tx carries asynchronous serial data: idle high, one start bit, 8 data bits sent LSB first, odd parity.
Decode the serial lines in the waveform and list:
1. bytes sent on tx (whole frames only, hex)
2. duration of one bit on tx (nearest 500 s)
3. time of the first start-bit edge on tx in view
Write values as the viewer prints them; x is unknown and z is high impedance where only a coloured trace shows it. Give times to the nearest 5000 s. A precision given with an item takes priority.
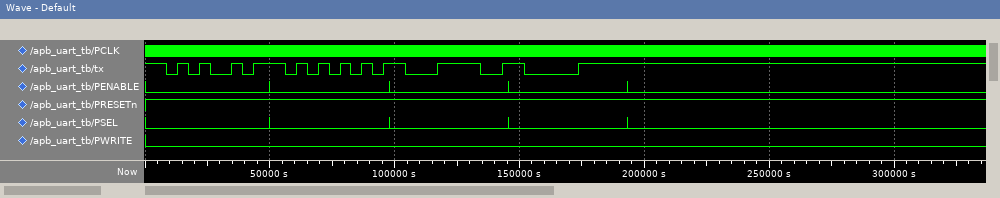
A5, 55, 3C, F0
4500 s
10000 s
